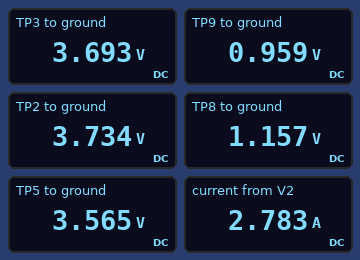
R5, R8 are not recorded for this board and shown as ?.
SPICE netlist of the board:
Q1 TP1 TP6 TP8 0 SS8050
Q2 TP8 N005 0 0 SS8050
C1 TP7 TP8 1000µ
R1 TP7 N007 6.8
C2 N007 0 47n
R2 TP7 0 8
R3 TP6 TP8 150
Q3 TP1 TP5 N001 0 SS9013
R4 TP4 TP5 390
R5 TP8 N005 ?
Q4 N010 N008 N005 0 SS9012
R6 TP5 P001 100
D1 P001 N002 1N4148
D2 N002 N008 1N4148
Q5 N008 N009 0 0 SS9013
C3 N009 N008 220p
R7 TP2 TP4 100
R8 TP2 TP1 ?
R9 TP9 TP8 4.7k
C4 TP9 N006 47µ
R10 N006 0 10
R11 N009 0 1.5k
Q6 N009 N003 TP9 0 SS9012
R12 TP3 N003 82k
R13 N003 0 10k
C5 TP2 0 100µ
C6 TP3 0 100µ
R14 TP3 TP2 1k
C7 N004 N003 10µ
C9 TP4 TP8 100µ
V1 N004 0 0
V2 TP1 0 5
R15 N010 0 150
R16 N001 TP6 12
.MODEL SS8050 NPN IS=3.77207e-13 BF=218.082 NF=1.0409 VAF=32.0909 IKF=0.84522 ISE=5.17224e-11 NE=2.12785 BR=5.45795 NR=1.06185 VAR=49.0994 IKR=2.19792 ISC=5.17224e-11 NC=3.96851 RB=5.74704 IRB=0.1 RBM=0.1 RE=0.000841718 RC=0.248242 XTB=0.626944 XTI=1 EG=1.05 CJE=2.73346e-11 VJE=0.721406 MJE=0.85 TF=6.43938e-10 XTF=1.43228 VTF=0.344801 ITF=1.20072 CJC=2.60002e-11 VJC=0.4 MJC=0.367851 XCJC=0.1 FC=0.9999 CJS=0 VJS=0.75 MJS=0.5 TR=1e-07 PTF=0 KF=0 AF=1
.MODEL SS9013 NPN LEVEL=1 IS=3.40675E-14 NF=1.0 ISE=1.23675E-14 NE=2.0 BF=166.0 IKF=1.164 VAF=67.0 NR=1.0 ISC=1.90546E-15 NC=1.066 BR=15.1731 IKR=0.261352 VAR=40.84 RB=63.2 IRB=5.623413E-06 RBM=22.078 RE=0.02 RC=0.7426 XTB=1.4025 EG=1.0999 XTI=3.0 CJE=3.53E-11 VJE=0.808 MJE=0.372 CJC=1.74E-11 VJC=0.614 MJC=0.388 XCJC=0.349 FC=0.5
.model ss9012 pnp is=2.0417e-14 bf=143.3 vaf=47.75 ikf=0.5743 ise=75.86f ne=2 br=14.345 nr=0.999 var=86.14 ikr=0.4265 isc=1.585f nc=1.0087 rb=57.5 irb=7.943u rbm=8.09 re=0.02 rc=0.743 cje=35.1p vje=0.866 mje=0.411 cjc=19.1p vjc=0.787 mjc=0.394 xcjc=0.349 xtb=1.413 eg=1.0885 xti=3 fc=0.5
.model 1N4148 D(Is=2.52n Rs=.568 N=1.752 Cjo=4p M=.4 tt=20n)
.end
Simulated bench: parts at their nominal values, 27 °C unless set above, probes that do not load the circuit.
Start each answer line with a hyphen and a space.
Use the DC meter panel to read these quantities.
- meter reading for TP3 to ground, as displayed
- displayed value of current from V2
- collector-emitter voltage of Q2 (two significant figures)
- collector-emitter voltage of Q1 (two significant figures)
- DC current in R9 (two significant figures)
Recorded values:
- 3.693 V
- 2.783 A
- 1.2 V
- 3.8 V
- 42 µA
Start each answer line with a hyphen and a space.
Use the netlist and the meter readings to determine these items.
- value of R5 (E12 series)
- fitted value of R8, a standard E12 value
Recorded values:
- 2.2 Ω
- 3.3 kΩ
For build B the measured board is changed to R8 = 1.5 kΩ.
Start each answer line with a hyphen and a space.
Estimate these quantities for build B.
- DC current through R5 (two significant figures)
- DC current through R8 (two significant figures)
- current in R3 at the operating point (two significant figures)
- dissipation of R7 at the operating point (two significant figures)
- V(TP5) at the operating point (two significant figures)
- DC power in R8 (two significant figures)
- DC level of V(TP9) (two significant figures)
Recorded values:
- 77 mA
- 520 µA
- 7.1 mA
- 23 µW
- 4.0 V
- 410 µW
- 1.0 V
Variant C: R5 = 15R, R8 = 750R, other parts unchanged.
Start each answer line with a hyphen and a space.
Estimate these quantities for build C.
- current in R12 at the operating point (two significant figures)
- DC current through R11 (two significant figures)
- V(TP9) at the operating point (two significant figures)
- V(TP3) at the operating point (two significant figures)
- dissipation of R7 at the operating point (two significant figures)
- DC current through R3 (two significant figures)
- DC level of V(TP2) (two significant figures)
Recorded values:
- 50 µA
- 180 µA
- 1.1 V
- 4.6 V
- 16 µW
- 6.9 mA
- 4.7 V
